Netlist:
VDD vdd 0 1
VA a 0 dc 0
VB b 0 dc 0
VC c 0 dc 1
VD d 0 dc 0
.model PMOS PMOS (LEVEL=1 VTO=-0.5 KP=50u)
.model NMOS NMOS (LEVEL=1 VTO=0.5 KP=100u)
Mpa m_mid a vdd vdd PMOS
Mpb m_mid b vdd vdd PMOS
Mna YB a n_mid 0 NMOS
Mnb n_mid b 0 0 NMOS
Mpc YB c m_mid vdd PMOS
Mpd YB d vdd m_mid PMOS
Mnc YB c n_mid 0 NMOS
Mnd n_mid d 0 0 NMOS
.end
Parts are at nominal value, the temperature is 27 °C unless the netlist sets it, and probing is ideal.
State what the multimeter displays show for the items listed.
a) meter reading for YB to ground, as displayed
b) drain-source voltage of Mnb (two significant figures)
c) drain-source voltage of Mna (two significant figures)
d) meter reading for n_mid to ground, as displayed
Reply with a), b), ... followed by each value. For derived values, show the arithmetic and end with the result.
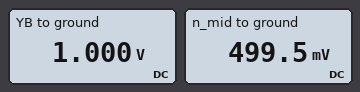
a) 1.000 V
b) 499.5 mV = 500 mV
c) 1 V - 499.5 mV = 500 mV
d) 499.5 mV
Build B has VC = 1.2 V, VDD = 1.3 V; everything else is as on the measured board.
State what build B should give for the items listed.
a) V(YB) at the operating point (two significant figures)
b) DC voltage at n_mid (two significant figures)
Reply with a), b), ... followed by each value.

a) 1.3 V
b) 700 mV
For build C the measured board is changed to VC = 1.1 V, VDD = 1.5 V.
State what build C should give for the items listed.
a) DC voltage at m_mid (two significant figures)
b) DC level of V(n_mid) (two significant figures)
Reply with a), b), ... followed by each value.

a) 1.5 V
b) 600 mV
